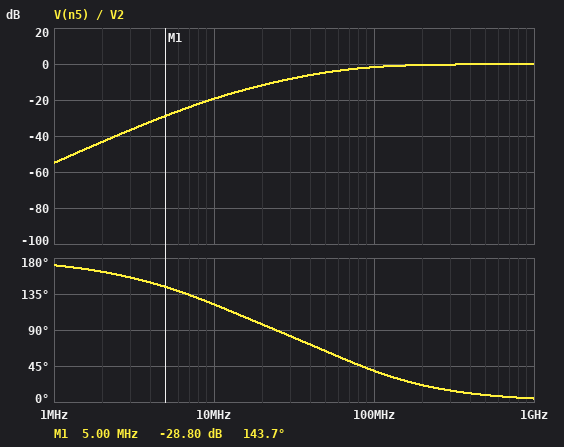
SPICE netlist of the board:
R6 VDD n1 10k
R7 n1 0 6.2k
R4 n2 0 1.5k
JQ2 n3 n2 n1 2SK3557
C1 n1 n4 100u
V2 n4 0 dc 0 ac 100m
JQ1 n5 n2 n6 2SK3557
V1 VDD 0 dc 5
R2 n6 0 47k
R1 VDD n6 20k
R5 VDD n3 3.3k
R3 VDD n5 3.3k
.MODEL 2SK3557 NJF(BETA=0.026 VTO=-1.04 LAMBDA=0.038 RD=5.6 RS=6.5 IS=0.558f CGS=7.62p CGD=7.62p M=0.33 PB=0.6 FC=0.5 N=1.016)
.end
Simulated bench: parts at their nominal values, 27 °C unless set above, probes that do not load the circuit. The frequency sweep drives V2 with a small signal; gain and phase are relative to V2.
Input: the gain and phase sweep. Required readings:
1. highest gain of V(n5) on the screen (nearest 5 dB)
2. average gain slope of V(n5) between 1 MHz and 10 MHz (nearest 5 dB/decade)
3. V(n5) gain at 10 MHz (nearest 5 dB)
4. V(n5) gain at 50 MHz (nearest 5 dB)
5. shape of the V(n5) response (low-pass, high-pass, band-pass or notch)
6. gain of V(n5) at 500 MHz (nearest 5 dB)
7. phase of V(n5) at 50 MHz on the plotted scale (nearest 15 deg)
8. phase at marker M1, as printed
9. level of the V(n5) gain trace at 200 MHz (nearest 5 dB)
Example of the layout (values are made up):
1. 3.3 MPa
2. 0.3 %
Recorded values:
1. 0 dB
2. 35 dB/decade
3. -20 dB
4. -5 dB
5. high-pass
6. 0 dB
7. 60 deg
8. 143.7 deg
9. 0 dB
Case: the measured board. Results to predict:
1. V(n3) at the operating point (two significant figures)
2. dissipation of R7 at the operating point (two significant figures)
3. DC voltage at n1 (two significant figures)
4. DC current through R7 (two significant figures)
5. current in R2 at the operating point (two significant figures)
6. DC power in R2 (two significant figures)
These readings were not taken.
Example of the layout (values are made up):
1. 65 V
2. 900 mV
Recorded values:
1. 5.0 V
2. 590 µW
3. 1.9 V
4. 310 µA
5. 75 µA
6. 260 µW
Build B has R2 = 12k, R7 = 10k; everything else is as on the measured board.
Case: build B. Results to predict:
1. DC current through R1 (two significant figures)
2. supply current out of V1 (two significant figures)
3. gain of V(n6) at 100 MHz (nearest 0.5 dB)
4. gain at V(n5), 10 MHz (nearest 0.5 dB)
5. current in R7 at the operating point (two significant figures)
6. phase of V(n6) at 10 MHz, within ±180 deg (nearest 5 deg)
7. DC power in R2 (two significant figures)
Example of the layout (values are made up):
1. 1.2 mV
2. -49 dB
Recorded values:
1. 160 µA
2. 410 µA
3. -2.0 dB
4. -20.5 dB
5. 250 µA
6. 90 deg
7. 290 µW
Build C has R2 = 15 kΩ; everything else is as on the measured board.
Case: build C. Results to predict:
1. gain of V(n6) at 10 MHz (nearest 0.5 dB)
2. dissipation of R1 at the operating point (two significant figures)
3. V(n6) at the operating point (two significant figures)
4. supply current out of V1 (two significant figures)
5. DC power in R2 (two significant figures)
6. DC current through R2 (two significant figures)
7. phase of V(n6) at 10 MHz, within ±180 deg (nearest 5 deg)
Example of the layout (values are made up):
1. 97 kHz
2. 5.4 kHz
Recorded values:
1. -14.0 dB
2. 410 µW
3. 2.1 V
4. 450 µA
5. 310 µW
6. 140 µA
7. 85 deg
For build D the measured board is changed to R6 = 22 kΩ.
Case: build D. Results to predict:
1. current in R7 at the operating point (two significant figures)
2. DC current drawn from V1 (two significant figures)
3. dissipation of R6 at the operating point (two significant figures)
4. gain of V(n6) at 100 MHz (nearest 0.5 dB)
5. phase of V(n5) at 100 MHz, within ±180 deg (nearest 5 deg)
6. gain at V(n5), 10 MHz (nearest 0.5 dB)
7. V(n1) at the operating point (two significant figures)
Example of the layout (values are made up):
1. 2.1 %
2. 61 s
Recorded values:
1. 180 µA
2. 250 µA
3. 690 µW
4. -1.0 dB
5. 35 deg
6. -18.0 dB
7. 1.1 V
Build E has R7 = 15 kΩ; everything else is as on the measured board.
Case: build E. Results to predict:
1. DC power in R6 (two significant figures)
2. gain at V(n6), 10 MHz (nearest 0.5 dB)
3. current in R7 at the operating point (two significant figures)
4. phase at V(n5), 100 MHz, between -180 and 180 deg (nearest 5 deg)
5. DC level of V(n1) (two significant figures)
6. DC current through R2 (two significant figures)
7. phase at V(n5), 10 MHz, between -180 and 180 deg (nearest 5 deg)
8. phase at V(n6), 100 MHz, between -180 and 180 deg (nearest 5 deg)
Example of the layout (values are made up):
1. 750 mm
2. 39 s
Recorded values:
1. 400 µW
2. -14.5 dB
3. 200 µA
4. 45 deg
5. 3.0 V
6. 75 µA
7. 125 deg
8. 35 deg
